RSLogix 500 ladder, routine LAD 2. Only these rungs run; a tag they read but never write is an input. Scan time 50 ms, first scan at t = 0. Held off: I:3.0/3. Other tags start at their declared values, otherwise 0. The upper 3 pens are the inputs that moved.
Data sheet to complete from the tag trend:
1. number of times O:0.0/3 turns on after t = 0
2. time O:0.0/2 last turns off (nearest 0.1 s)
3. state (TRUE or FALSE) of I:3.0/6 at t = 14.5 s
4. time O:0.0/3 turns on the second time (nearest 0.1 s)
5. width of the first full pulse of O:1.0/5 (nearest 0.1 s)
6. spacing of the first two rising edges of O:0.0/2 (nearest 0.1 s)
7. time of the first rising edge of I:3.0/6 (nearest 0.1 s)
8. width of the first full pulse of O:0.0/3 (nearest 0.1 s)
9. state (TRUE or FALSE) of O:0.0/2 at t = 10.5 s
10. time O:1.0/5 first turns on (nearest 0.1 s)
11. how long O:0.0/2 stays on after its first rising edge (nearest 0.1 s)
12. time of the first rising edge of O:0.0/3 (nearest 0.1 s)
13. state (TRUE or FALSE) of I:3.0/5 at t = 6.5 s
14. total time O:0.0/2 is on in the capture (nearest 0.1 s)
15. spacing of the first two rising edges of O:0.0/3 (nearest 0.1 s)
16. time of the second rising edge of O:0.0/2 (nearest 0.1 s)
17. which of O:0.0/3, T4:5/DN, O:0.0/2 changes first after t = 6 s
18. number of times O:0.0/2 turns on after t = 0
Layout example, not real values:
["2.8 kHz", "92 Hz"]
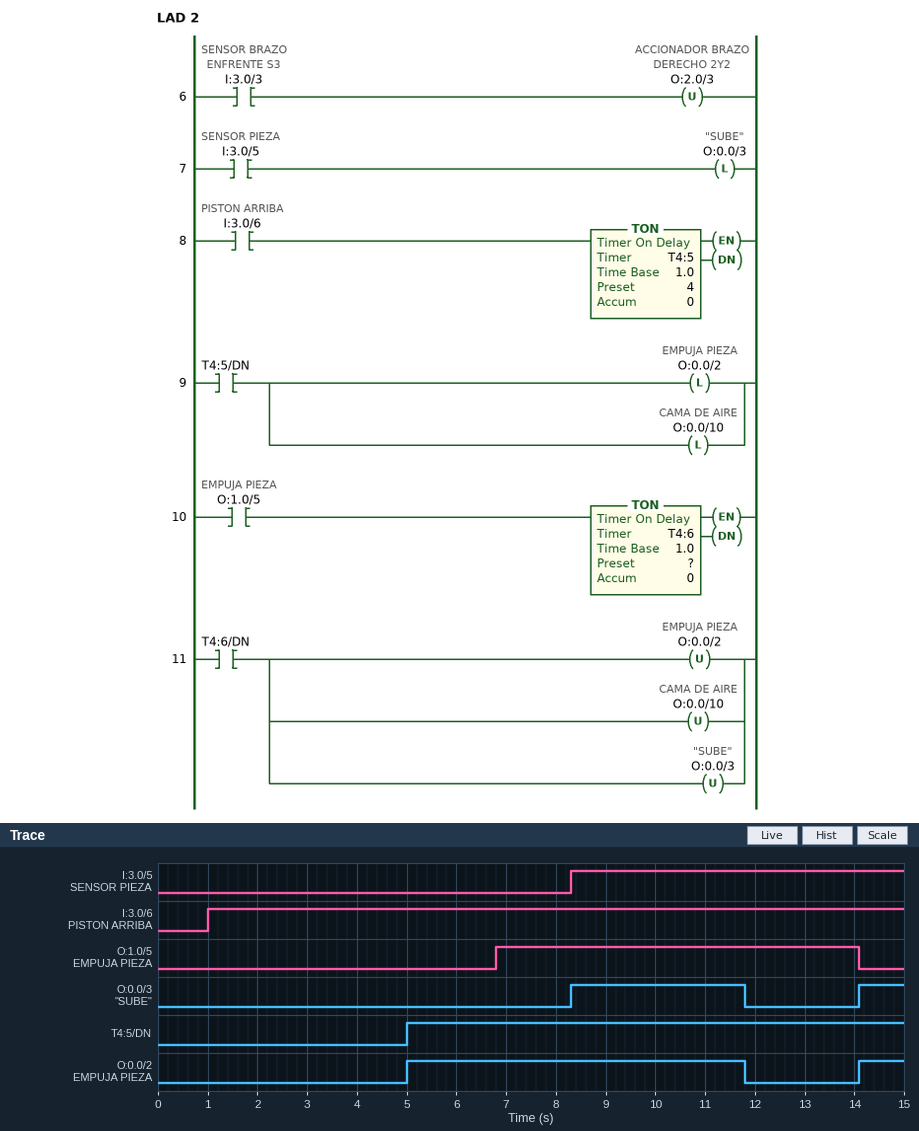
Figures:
["2", "11.8 s", "TRUE", "14.1 s", "7.3 s", "9.1 s", "1.0 s", "3.5 s", "TRUE", "6.8 s", "6.8 s", "8.3 s", "FALSE", "7.7 s", "5.8 s", "14.1 s", "O:0.0/3", "2"]
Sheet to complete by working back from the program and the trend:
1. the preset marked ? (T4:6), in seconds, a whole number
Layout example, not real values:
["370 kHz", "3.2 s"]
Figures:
["5 s"]
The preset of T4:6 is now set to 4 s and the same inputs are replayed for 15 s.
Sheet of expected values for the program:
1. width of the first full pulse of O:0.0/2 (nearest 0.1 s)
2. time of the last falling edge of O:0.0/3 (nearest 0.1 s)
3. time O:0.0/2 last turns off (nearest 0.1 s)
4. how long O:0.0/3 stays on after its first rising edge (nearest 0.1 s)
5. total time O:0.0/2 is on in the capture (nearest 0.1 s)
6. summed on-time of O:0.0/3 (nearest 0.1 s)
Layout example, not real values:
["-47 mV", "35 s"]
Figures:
["5.8 s", "10.8 s", "10.8 s", "2.5 s", "6.7 s", "3.4 s"]
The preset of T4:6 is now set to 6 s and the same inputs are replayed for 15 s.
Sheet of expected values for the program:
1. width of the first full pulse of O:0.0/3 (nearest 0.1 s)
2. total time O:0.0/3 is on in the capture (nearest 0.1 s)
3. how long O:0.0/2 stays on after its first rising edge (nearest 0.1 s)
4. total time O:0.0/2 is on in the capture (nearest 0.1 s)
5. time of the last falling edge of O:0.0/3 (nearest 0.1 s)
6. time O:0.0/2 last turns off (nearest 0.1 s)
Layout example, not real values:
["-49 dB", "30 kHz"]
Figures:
["4.5 s", "5.4 s", "7.8 s", "8.7 s", "12.8 s", "12.8 s"]
